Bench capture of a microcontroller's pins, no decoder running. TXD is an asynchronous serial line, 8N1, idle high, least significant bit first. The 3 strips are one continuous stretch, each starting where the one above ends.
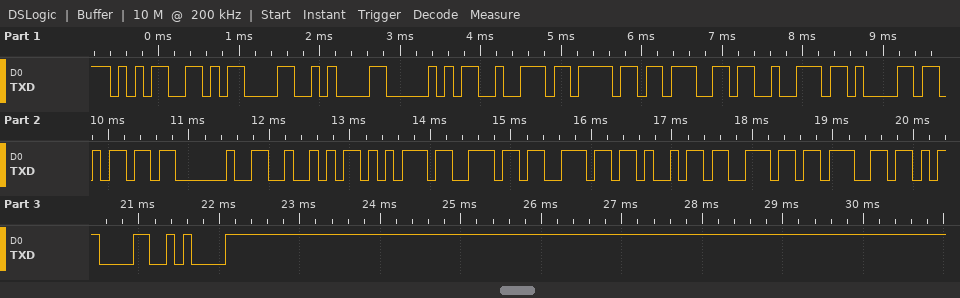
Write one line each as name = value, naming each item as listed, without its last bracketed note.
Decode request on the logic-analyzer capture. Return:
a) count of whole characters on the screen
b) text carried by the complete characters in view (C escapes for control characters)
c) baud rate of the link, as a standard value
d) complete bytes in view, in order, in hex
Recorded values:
count of whole characters on the screen = 20
text carried by the complete characters in view = "5\r\nProgram Running\r\n"
baud rate of the link, as a standard value = 9600 baud
complete bytes in view, in order, in hex = 35 0D 0A 50 72 6F 67 72 61 6D 20 52 75 6E 6E 69 6E 67 0D 0A
